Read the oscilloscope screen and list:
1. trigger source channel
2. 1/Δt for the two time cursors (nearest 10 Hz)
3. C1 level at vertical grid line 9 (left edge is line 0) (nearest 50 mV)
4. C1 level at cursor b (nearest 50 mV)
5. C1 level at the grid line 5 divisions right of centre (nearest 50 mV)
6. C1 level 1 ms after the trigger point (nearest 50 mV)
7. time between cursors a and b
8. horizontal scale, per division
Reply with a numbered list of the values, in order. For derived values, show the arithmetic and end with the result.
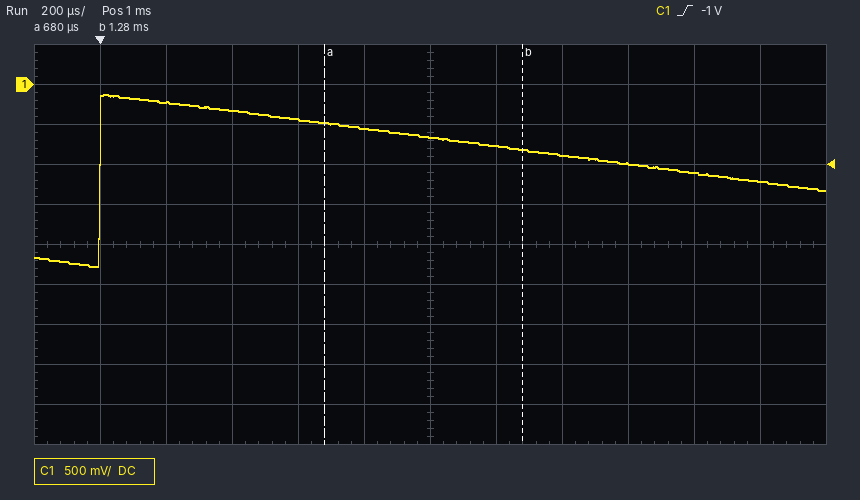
1. C1
2. 1 / 600 µs ≈ 1.67 kHz
3. -1.00 V
4. -800 mV
5. -1.20 V
6. -650 mV
7. 1.28 ms − (680 µs) = 600 µs
8. 200 µs
